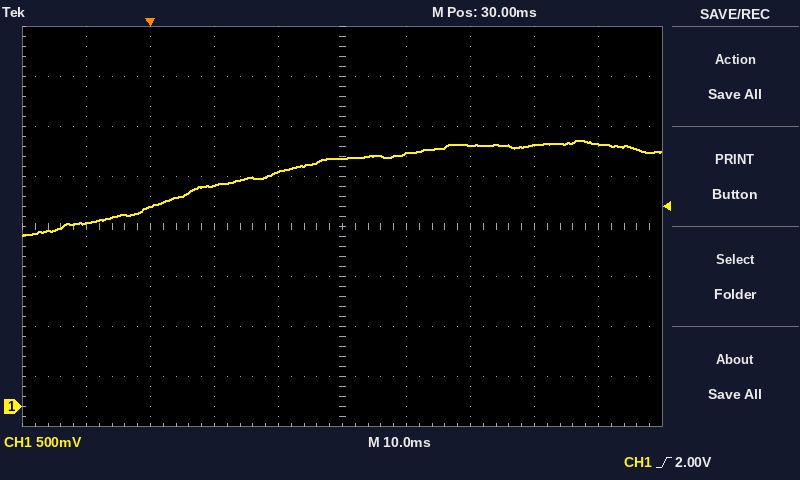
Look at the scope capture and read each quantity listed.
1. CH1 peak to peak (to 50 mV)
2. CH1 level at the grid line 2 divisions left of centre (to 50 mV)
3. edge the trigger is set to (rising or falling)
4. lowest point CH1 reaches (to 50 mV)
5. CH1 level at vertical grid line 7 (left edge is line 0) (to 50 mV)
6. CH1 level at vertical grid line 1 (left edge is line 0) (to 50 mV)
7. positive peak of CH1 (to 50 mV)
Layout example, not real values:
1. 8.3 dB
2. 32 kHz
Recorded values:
1. 950 mV
2. 2.20 V
3. rising
4. 1.70 V
5. 2.60 V
6. 1.85 V
7. 2.65 V
